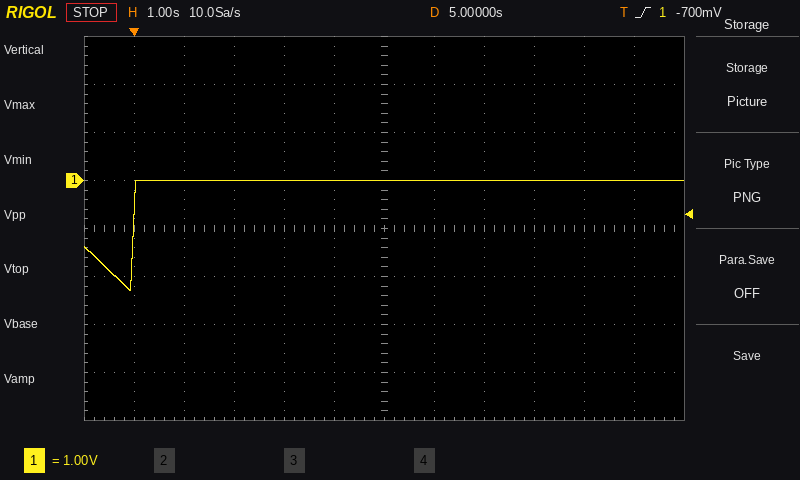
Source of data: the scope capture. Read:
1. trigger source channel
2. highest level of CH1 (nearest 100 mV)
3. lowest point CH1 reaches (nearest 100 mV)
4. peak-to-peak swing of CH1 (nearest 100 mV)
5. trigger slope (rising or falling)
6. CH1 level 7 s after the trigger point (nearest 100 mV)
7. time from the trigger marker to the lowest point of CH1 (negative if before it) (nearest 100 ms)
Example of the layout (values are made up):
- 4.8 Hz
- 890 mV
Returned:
- CH1
- 0.0 V
- -2.3 V
- 2.3 V
- rising
- 0.0 V
- -100 ms
